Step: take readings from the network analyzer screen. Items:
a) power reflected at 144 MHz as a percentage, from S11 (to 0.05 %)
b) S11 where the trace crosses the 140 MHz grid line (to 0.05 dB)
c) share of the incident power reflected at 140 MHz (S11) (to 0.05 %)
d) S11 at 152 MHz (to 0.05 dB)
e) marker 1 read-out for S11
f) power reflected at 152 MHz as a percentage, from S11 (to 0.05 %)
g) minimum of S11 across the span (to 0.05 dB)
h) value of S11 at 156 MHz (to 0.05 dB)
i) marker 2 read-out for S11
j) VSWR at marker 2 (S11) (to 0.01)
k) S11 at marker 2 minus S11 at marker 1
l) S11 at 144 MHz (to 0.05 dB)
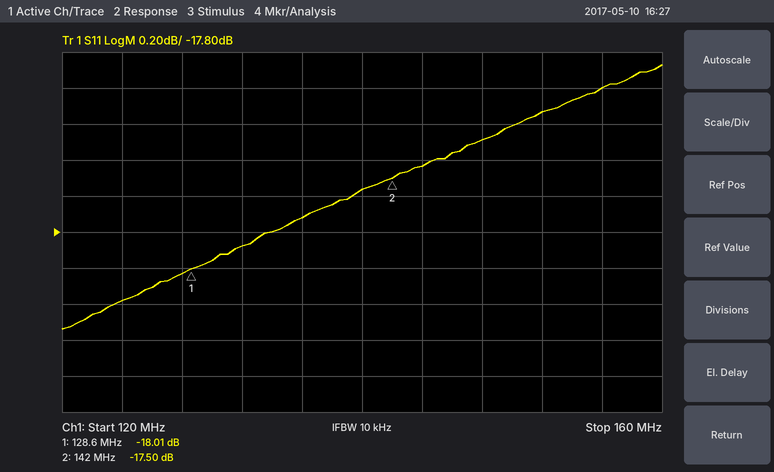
1.80 %
-17.55 dB
1.75 %
-17.15 dB
-18.01 dB
1.95 %
-18.35 dB
-17.00 dB
-17.50 dB
1.31
0.51 dB
-17.45 dB
